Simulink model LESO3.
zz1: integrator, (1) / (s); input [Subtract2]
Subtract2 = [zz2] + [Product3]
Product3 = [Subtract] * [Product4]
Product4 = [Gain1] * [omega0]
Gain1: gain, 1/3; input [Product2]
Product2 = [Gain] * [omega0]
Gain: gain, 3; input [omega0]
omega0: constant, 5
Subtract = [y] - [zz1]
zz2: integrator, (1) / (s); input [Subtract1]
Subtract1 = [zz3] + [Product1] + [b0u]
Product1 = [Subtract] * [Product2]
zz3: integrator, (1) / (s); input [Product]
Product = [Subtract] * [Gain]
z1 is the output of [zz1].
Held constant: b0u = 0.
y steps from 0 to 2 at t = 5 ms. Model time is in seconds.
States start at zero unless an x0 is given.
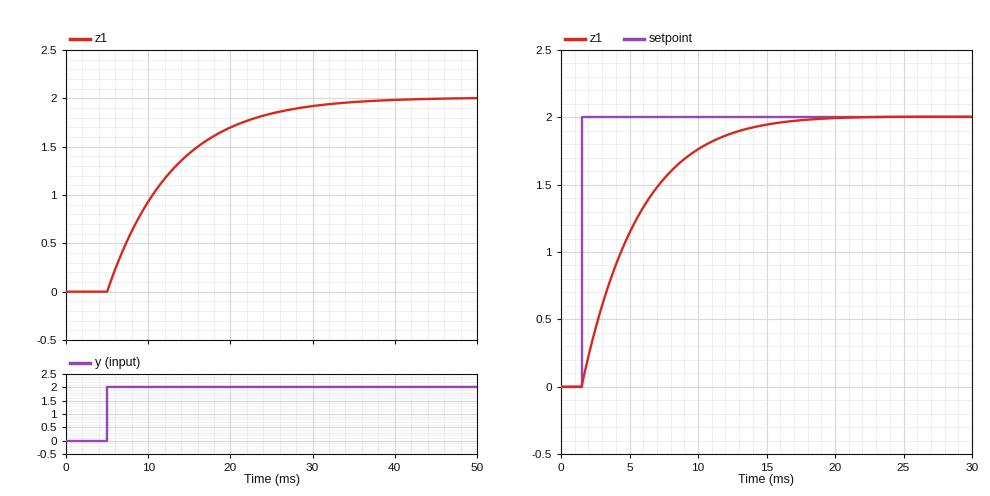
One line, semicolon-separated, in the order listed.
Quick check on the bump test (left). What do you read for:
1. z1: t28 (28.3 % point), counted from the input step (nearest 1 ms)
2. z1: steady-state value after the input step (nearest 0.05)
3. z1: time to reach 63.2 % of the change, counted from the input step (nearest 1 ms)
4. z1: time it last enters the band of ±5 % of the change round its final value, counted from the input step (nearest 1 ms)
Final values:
3 ms; 2.00; 8 ms; 24 ms
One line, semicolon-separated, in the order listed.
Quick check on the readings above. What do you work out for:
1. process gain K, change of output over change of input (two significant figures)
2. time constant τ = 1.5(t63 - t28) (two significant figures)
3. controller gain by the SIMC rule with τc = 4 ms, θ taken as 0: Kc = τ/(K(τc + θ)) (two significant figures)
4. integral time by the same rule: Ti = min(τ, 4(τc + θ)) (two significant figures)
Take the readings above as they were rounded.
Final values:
1.0; 7.5 ms; 1.9; 7.5 ms
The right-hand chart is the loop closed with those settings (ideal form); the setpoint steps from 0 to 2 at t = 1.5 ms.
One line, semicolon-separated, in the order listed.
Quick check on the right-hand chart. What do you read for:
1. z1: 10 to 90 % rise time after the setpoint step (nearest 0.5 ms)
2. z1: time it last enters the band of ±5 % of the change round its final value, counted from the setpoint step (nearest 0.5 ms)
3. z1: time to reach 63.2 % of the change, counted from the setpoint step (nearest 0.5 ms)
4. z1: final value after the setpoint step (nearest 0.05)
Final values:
8.5 ms; 11.5 ms; 4.0 ms; 2.00
